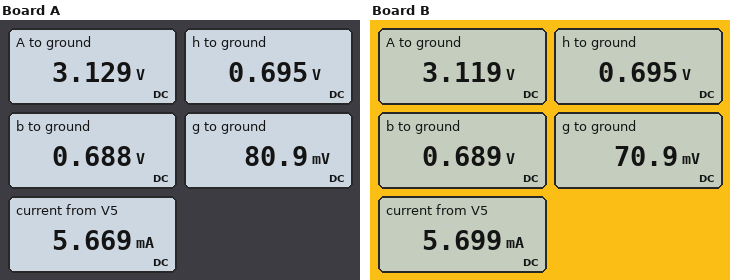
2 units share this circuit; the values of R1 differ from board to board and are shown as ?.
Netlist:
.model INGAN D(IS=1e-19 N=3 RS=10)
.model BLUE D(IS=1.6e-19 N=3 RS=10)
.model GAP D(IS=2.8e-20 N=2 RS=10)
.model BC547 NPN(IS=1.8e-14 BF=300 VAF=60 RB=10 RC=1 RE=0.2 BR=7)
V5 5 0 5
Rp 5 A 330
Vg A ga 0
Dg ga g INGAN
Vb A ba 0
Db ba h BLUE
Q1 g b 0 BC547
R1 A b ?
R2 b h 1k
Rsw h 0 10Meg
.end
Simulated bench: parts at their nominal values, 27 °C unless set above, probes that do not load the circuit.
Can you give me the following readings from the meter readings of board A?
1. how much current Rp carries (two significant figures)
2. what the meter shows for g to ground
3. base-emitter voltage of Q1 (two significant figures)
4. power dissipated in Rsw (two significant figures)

5.7 mA
80.9 mV
690 mV
48 nW
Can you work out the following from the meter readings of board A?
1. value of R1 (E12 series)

39 kΩ
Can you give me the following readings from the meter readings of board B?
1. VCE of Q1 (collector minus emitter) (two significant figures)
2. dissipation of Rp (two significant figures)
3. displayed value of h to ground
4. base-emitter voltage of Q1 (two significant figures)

71 mV
11 mW
0.695 V
690 mV
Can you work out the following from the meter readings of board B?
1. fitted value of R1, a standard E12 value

27 kΩ
